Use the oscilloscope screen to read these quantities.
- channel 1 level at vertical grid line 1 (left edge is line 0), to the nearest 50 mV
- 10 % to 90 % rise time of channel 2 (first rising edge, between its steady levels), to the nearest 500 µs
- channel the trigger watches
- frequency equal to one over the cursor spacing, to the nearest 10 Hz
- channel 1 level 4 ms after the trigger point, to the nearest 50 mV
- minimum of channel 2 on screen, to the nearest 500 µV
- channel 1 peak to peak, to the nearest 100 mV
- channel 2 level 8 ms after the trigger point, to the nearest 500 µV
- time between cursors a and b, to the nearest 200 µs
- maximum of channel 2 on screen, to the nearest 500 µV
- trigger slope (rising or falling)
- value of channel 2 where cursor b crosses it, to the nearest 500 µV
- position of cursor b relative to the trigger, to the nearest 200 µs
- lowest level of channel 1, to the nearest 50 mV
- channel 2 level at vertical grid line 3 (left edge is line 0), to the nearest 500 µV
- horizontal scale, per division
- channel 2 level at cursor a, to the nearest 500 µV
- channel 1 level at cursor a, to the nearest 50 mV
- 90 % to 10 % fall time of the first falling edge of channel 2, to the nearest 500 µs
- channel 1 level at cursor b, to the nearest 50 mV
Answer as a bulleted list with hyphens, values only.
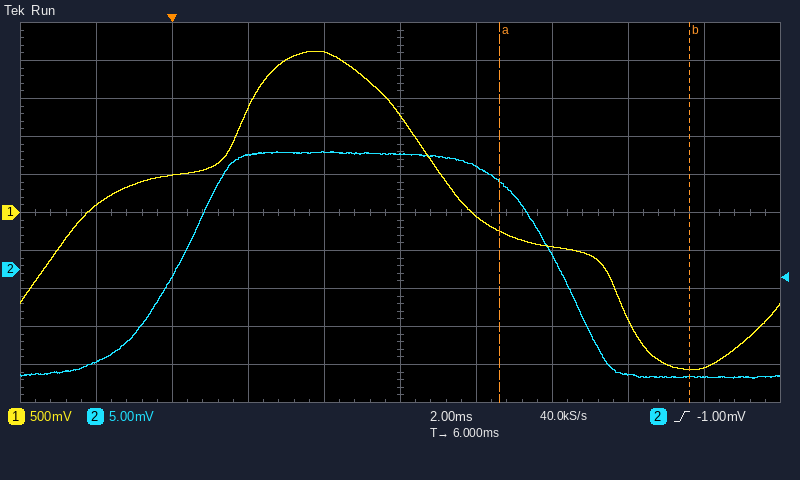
- 100 mV
- 3.0 ms
- channel 2
- 200 Hz
- 2.10 V
- -14.5 mV
- 4.20 V
- 13.5 mV
- 5.0 ms
- 15.5 mV
- rising
- -14.0 mV
- +13.6 ms
- -2.05 V
- 15.0 mV
- 2 ms
- 11.5 mV
- -250 mV
- 3.0 ms
- -2.05 V
